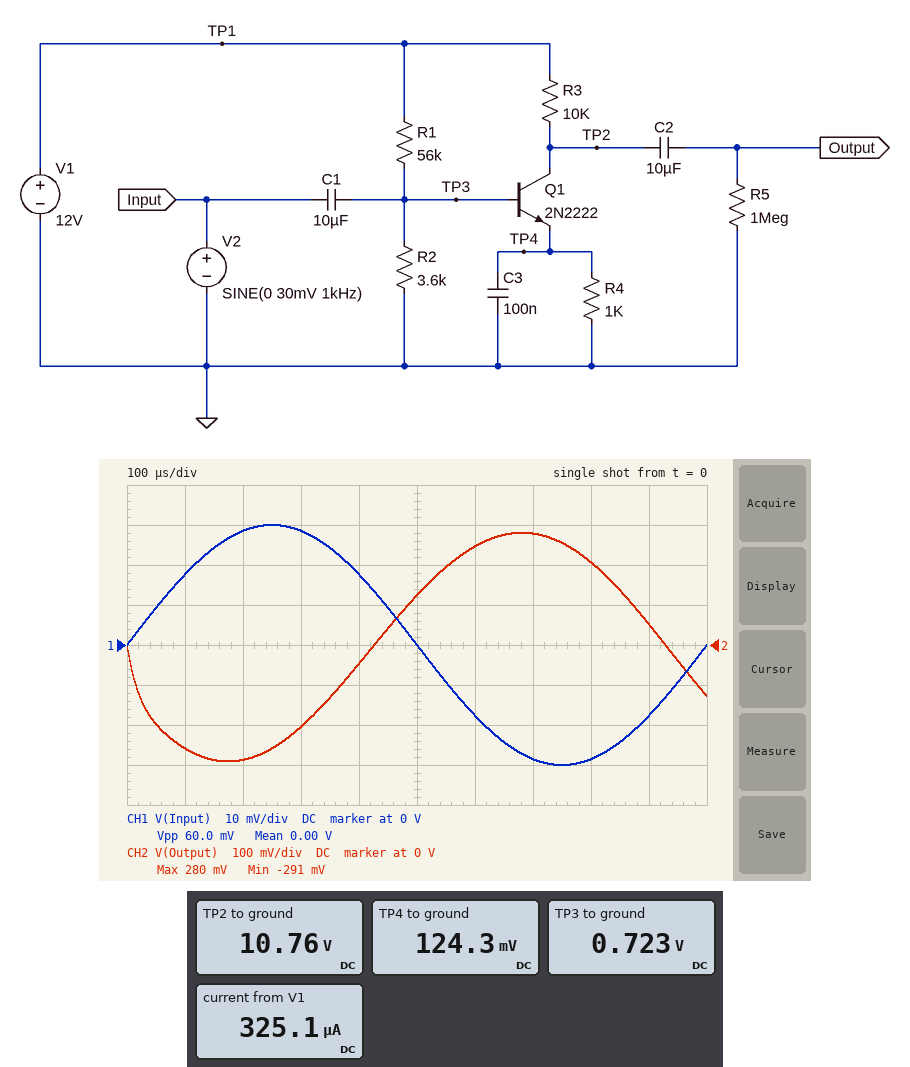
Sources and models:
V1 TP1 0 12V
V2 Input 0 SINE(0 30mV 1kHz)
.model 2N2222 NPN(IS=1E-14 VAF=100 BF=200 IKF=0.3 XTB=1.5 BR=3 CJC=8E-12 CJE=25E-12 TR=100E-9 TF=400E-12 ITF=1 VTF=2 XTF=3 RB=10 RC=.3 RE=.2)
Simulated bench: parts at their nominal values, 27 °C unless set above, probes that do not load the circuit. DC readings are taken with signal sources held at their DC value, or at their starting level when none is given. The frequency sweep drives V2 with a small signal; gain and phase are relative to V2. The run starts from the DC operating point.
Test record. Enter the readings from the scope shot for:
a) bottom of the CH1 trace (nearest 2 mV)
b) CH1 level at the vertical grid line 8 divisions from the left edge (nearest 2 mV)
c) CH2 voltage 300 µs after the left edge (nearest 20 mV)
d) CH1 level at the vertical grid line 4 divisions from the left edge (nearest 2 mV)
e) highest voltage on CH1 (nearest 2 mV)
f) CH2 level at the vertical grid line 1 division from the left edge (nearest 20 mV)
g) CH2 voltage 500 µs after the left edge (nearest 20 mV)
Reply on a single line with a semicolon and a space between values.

-30 mV; -28 mV; -200 mV; 18 mV; 30 mV; -260 mV; 120 mV
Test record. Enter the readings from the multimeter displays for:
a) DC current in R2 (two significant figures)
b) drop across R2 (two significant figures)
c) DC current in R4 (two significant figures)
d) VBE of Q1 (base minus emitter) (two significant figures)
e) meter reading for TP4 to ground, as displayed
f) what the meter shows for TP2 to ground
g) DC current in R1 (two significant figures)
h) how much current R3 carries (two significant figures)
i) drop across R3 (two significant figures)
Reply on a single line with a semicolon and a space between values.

200 µA; 720 mV; 120 µA; 600 mV; 124.3 mV; 10.76 V; 200 µA; 120 µA; 1.2 V
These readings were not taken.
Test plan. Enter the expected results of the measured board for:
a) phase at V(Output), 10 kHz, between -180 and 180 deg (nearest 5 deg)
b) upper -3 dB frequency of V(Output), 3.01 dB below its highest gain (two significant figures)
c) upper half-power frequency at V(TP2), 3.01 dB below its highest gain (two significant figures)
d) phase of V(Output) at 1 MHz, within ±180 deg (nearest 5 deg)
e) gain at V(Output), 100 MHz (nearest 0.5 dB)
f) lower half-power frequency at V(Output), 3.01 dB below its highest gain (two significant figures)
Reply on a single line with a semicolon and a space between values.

-145 deg; 4.7 MHz; 4.7 MHz; 170 deg; 7.5 dB; 8.8 kHz
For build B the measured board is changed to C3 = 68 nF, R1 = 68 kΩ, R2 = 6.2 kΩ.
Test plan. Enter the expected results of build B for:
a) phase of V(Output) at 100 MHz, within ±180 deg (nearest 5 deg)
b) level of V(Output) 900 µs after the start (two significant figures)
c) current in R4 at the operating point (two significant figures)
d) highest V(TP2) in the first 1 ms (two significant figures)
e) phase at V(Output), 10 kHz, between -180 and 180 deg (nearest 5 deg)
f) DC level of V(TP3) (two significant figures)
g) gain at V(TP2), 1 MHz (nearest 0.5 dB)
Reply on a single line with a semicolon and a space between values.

70 deg; 75 mV; 370 µA; 8.7 V; -120 deg; 990 mV; 42.5 dB
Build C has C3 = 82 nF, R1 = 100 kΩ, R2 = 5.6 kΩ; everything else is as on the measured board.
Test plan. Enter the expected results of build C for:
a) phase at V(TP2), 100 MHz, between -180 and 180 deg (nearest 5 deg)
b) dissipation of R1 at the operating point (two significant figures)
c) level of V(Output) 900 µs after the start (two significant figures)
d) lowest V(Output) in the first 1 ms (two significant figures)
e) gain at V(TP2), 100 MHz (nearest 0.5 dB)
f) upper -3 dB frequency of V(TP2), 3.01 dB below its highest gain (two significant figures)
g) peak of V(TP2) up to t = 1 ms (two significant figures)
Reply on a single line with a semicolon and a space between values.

35 deg; 1.3 mW; 72 mV; -240 mV; 3.0 dB; 4.9 MHz; 12 V
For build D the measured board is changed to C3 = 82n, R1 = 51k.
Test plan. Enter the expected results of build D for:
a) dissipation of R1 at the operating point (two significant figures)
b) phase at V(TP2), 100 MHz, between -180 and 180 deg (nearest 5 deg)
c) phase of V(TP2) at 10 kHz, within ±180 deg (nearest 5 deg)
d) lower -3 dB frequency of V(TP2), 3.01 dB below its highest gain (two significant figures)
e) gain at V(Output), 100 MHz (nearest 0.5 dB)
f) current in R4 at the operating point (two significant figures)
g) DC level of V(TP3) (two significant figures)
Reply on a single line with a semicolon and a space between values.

2.5 mW; 60 deg; -135 deg; 15 kHz; 10.0 dB; 180 µA; 790 mV
